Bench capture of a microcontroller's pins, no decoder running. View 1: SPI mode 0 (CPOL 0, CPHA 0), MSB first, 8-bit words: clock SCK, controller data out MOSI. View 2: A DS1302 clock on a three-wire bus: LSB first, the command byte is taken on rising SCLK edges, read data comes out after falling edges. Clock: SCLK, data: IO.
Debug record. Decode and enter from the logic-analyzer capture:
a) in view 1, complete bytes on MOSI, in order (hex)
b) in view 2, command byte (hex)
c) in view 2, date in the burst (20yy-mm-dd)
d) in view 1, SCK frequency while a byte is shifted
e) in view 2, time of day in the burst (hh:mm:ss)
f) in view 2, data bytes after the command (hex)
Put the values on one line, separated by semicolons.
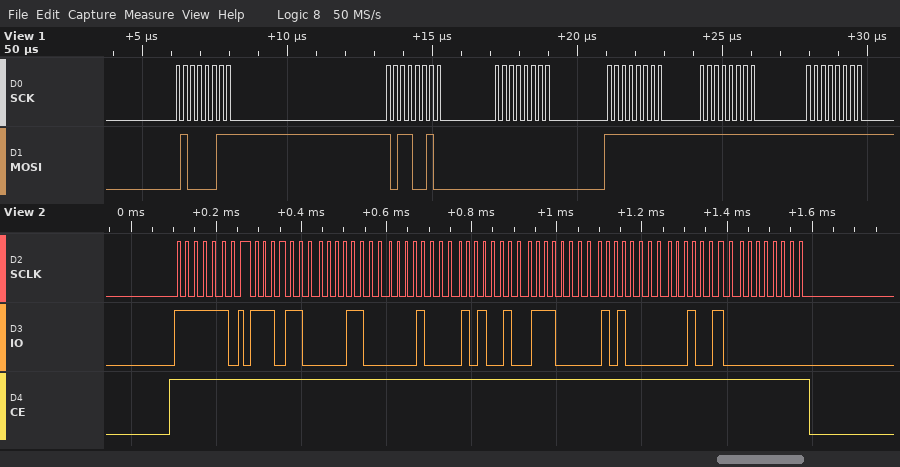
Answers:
43 B2 00 FF FF FF; 0xBF; 2024-07-25; 4 MHz; 08:18:37; 37 18 08 25 07 05 24 00
